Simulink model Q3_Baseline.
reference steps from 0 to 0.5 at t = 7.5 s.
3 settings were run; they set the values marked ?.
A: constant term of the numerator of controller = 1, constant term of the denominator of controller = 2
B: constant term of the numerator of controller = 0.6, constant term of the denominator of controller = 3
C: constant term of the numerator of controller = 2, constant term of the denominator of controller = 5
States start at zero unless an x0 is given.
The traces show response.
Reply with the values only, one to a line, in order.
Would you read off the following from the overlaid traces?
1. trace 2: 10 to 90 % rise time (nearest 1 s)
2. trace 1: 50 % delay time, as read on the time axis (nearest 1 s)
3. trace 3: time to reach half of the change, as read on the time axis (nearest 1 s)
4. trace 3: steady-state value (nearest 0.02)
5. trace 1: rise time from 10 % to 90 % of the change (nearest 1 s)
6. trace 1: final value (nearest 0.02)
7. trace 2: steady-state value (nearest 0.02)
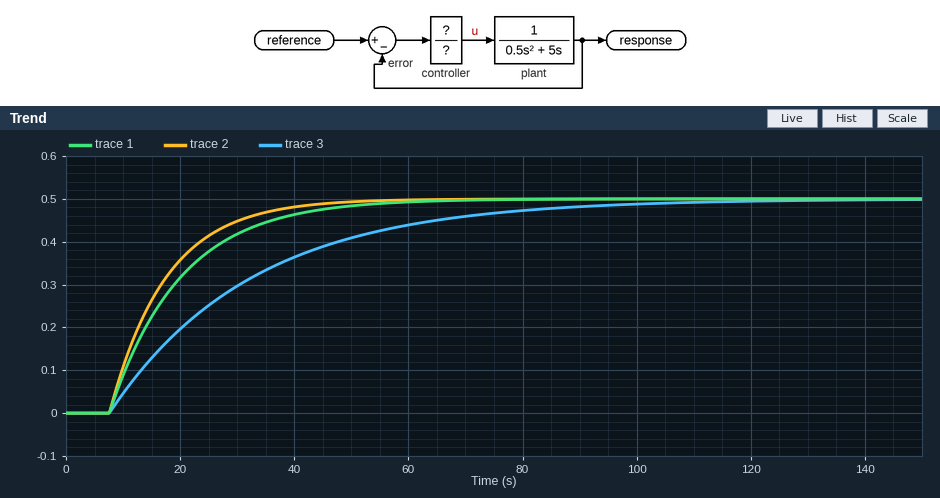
22 s
16 s
25 s
0.50
27 s
0.50
0.50
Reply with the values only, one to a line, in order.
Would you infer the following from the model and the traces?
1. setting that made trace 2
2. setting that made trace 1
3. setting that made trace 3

A
C
B
